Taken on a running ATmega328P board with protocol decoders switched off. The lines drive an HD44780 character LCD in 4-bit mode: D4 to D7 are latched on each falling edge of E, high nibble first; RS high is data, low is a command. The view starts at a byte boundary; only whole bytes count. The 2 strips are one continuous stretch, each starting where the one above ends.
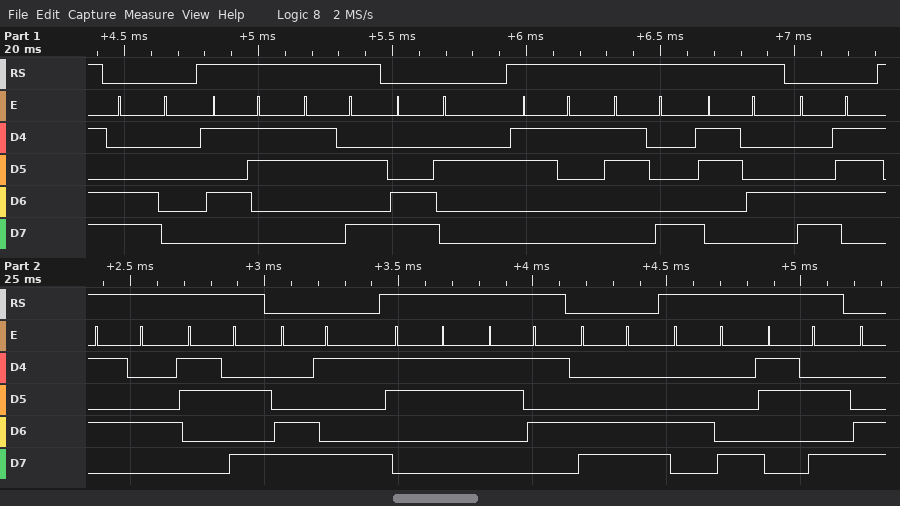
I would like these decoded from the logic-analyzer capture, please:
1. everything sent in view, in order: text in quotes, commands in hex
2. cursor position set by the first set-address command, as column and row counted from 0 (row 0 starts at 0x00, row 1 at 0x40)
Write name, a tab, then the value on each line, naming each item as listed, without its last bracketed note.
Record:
everything sent in view, in order: text in quotes, commands in hex	0xC0 "S:" 0xC2 "184" 0xC7 "T:" 0xC9 "35" 0xCC "H:"
cursor position set by the first set-address command, as column and row counted from 0	column 0, row 1
